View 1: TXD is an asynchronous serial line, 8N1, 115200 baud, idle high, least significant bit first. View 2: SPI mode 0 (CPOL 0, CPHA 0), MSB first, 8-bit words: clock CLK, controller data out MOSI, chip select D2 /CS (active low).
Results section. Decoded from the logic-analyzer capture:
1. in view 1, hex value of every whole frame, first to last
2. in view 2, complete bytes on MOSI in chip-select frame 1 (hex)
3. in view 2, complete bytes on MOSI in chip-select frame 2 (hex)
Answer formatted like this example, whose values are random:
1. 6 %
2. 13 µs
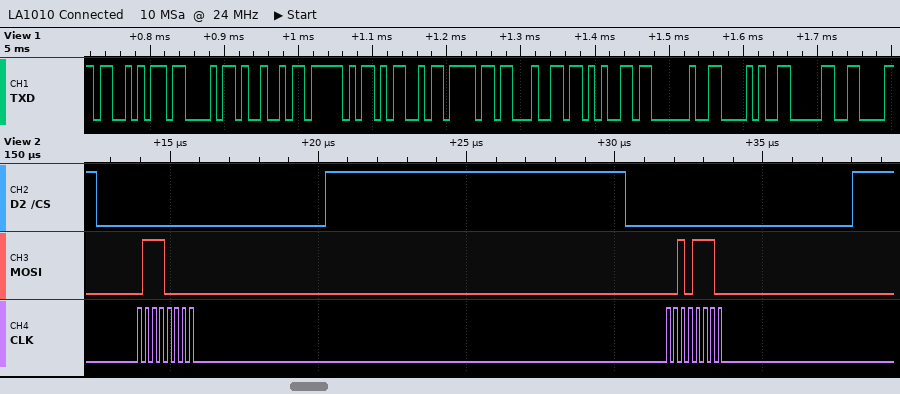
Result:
1. 53 43 49 5F 4D 6F 64 65 20 28 30
2. 70
3. 2E
